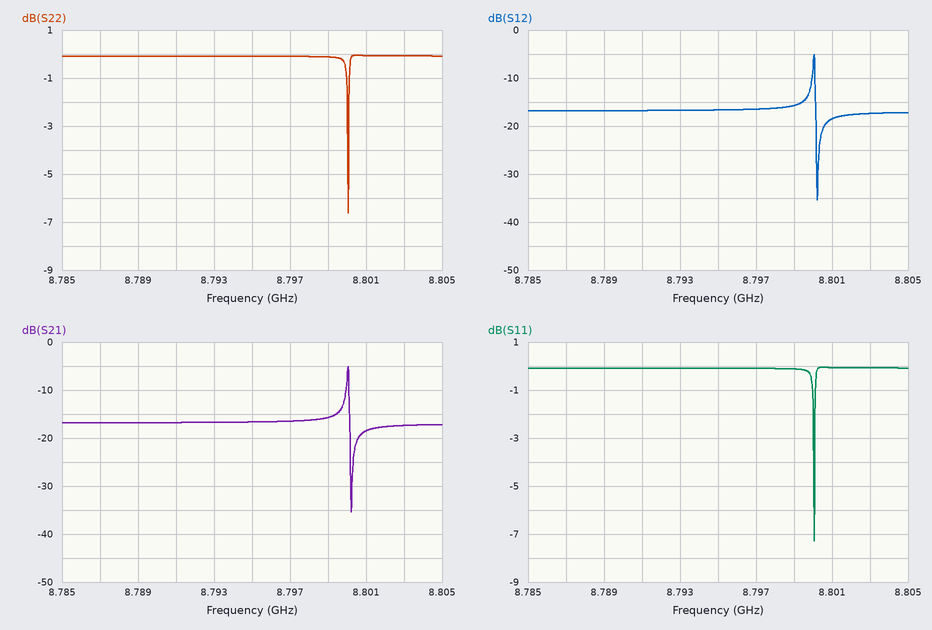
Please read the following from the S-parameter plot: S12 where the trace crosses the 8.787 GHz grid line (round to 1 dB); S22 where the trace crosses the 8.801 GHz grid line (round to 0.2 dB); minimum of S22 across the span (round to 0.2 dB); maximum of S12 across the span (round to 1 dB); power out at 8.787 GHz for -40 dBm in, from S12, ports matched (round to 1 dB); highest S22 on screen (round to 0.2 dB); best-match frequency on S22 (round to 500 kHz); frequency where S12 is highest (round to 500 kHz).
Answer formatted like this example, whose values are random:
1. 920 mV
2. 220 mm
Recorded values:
1. -17 dB
2. 0.0 dB
3. -6.6 dB
4. -5 dB
5. -57 dBm
6. 0.0 dB
7. 8.8000 GHz
8. 8.8000 GHz
